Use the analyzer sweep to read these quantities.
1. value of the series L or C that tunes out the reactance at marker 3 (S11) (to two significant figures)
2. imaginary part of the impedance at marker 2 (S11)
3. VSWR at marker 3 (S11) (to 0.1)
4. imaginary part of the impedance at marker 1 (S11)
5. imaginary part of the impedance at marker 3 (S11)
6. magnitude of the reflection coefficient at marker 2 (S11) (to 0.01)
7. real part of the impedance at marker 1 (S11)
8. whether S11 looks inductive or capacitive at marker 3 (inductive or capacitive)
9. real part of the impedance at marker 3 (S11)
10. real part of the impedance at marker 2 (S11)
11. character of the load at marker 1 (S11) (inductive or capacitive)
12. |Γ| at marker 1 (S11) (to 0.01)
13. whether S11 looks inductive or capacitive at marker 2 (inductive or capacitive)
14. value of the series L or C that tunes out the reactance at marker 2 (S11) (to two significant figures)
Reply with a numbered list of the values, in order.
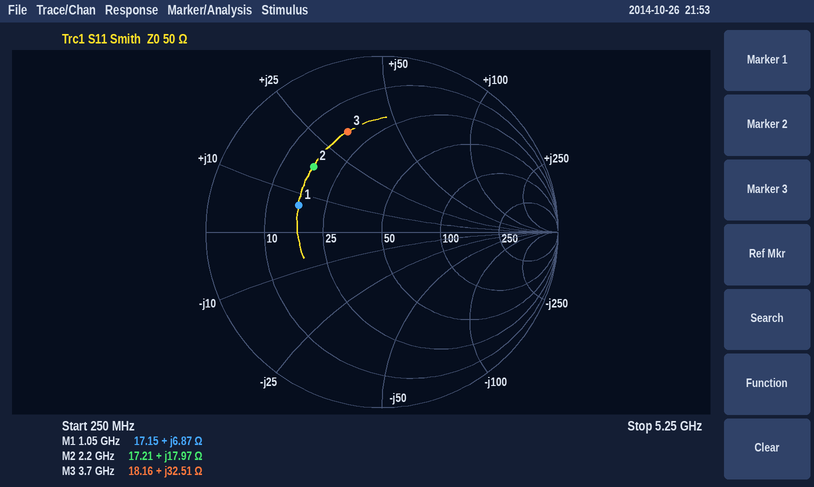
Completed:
1. 1.3 pF
2. +17.97 Ω
3. 4.0
4. +6.87 Ω
5. +32.51 Ω
6. 0.54
7. 17.15 Ω
8. inductive
9. 18.16 Ω
10. 17.21 Ω
11. inductive
12. 0.50
13. inductive
14. 4.0 pF
